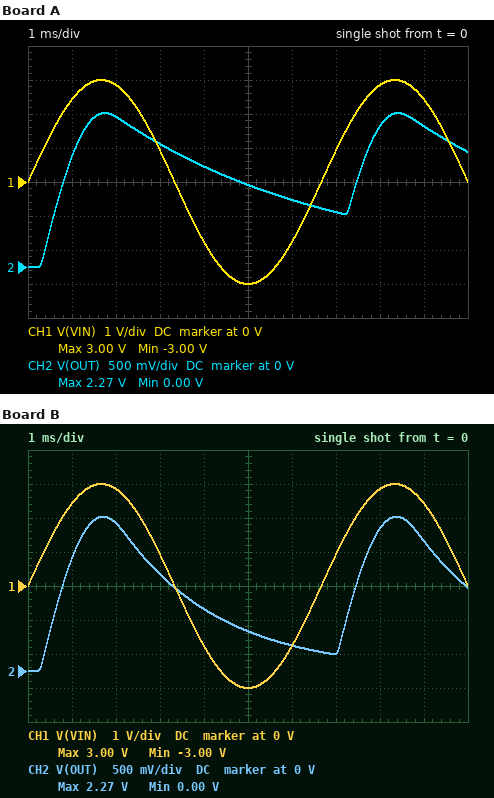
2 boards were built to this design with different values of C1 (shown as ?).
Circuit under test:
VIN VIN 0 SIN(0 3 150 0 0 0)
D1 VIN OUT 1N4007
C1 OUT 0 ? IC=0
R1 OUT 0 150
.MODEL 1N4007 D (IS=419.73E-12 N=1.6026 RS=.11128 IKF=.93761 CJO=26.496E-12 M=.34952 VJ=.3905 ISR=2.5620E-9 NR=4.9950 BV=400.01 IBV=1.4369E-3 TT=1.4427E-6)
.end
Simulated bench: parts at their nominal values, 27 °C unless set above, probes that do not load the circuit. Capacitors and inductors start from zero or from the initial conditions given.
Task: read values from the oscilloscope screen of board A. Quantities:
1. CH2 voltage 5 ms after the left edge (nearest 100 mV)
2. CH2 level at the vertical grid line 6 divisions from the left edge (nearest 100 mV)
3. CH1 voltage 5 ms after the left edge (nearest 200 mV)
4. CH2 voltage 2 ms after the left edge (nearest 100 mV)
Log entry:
1.2 V
1.0 V
-3.0 V
2.2 V
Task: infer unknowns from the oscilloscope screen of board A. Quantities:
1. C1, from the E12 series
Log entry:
33 µF
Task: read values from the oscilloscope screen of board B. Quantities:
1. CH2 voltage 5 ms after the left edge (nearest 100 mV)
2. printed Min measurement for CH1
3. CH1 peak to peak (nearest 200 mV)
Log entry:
600 mV
-3.00 V
6.0 V
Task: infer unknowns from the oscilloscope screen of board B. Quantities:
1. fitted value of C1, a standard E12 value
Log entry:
15 µF
